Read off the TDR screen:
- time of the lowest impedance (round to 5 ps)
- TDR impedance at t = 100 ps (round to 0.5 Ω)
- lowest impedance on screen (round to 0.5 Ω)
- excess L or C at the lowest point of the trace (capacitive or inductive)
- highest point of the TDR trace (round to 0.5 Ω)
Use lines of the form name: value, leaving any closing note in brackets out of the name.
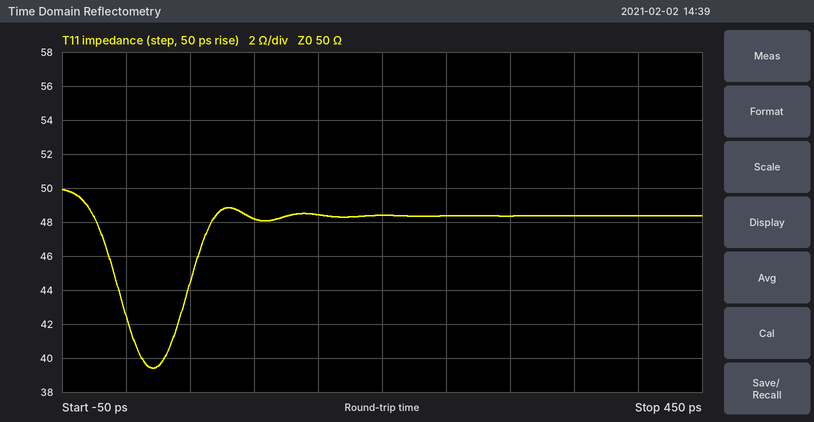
time of the lowest impedance: 20 ps
TDR impedance at t = 100 ps: 48.0 Ω
lowest impedance on screen: 39.5 Ω
excess L or C at the lowest point of the trace: capacitive
highest point of the TDR trace: 50.0 Ω
